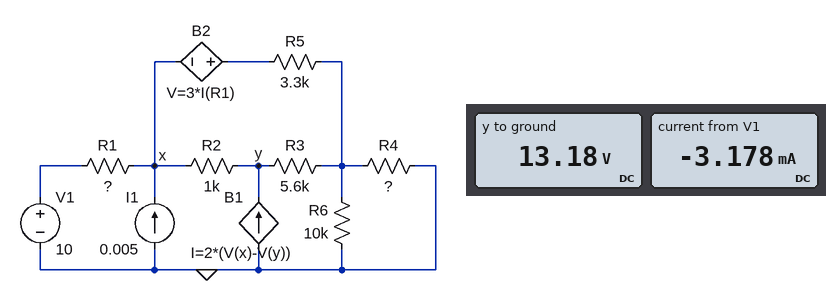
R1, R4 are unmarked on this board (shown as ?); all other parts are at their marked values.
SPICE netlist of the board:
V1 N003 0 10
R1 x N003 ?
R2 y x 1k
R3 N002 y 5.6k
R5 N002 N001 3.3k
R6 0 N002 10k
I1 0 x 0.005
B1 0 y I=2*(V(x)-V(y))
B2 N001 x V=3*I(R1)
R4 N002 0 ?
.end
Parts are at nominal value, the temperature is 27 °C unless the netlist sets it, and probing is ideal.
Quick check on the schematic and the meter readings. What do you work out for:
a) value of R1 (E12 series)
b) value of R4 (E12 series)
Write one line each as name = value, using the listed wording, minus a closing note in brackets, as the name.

value of R1 = 1 kΩ
value of R4 = 3.3 kΩ
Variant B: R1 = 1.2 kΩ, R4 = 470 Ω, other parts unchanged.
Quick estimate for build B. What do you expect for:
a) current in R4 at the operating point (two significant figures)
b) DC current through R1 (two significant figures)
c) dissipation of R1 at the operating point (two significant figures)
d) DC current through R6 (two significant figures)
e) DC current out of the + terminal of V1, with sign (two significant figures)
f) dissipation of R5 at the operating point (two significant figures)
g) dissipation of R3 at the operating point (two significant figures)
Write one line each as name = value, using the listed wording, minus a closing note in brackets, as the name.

current in R4 at the operating point = 4.7 mA
DC current through R1 = 1.9 mA
dissipation of R1 at the operating point = 4.5 mW
DC current through R6 = 220 µA
DC current out of the + terminal of V1, with sign = -1.9 mA
dissipation of R5 at the operating point = 31 mW
dissipation of R3 at the operating point = 18 mW
